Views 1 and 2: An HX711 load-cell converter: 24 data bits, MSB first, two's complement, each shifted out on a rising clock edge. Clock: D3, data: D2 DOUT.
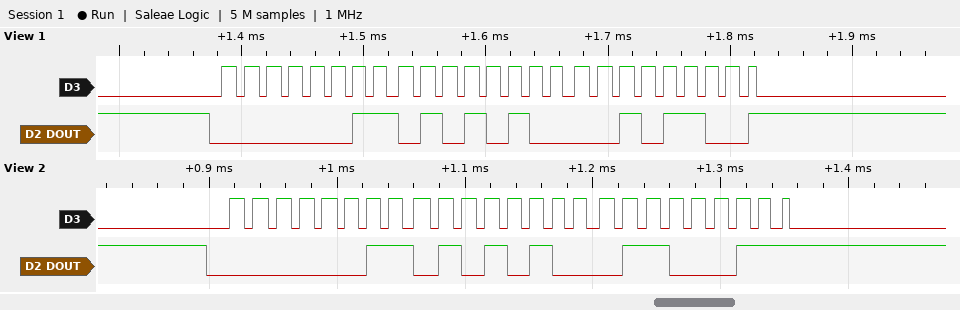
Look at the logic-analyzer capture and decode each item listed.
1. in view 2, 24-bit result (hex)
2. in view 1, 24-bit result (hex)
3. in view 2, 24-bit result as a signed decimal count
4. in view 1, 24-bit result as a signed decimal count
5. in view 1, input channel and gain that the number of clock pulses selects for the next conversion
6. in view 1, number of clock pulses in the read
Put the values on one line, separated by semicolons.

0x035463; 0x03542C; 218211; 218156; channel A, gain 128; 25
